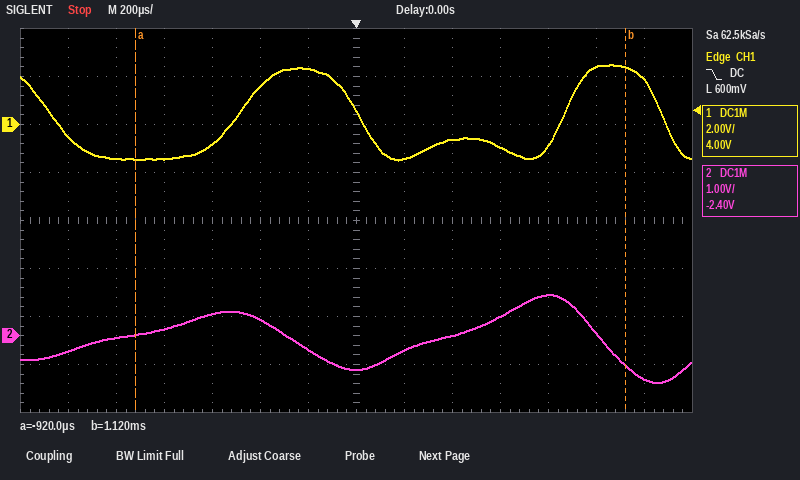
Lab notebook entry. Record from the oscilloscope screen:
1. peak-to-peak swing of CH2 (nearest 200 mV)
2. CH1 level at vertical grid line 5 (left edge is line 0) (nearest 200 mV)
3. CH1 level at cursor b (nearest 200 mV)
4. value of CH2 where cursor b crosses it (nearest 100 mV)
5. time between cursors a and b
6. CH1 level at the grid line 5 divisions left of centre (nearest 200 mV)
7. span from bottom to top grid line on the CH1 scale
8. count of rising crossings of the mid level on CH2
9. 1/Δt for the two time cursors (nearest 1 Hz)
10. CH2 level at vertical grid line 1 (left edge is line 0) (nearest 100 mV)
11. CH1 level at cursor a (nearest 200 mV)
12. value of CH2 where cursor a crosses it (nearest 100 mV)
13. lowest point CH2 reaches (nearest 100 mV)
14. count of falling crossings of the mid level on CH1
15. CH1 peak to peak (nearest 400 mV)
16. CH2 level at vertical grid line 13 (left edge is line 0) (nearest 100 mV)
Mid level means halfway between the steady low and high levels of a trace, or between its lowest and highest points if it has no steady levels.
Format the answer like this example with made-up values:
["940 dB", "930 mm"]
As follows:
["1.8 V", "1.6 V", "2.4 V", "-600 mV", "2.04 ms", "-1.4 V", "16 V", "2", "490 Hz", "-300 mV", "-1.4 V", "0.0 V", "-1.0 V", "3", "4.0 V", "-900 mV"]
